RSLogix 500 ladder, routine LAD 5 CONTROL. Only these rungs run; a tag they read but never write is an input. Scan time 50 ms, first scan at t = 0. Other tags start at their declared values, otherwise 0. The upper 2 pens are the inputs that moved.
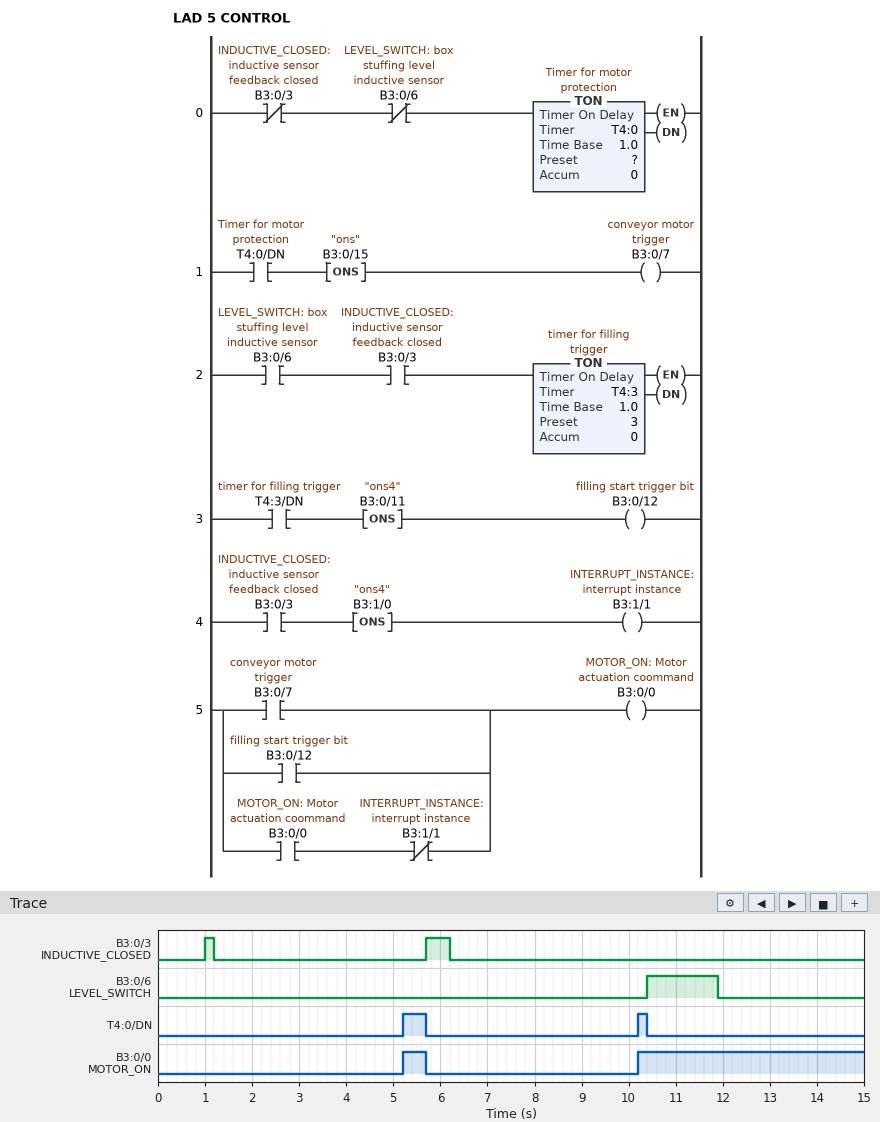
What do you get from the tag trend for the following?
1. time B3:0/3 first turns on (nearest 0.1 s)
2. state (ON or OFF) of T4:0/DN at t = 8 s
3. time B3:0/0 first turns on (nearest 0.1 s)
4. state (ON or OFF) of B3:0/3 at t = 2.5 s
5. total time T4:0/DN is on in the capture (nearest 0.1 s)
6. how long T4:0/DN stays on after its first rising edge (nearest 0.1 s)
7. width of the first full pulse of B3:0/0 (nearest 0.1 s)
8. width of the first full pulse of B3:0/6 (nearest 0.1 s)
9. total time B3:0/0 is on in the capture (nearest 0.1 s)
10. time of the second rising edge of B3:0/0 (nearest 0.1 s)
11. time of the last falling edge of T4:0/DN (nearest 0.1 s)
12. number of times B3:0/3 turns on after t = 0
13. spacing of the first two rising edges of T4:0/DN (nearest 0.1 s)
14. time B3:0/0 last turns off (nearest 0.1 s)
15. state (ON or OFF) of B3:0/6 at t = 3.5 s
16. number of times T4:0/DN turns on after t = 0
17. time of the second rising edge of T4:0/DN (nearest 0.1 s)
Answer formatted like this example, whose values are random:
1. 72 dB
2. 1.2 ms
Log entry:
1. 1.0 s
2. OFF
3. 5.2 s
4. OFF
5. 0.7 s
6. 0.5 s
7. 0.5 s
8. 1.5 s
9. 5.3 s
10. 10.2 s
11. 10.4 s
12. 2
13. 5.0 s
14. 5.7 s
15. OFF
16. 2
17. 10.2 s
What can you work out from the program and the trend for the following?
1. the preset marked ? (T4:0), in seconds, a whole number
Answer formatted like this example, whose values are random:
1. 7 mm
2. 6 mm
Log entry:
1. 4 s
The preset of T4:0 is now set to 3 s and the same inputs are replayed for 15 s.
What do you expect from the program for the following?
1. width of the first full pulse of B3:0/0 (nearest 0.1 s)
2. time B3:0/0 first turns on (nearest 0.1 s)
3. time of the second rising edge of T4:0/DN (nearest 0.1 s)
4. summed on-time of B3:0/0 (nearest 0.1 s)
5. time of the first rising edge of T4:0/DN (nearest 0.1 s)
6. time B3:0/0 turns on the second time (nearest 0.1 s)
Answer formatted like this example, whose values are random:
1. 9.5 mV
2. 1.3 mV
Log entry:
1. 1.5 s
2. 4.2 s
3. 9.2 s
4. 7.3 s
5. 4.2 s
6. 9.2 s
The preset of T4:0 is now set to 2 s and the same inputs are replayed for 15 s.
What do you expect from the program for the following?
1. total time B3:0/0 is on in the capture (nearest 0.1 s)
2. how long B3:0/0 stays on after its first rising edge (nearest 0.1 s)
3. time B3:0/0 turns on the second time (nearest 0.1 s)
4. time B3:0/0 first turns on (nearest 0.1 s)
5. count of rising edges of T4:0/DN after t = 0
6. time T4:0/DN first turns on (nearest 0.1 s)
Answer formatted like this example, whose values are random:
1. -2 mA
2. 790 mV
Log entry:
1. 9.3 s
2. 2.5 s
3. 8.2 s
4. 3.2 s
5. 3
6. 3.2 s
